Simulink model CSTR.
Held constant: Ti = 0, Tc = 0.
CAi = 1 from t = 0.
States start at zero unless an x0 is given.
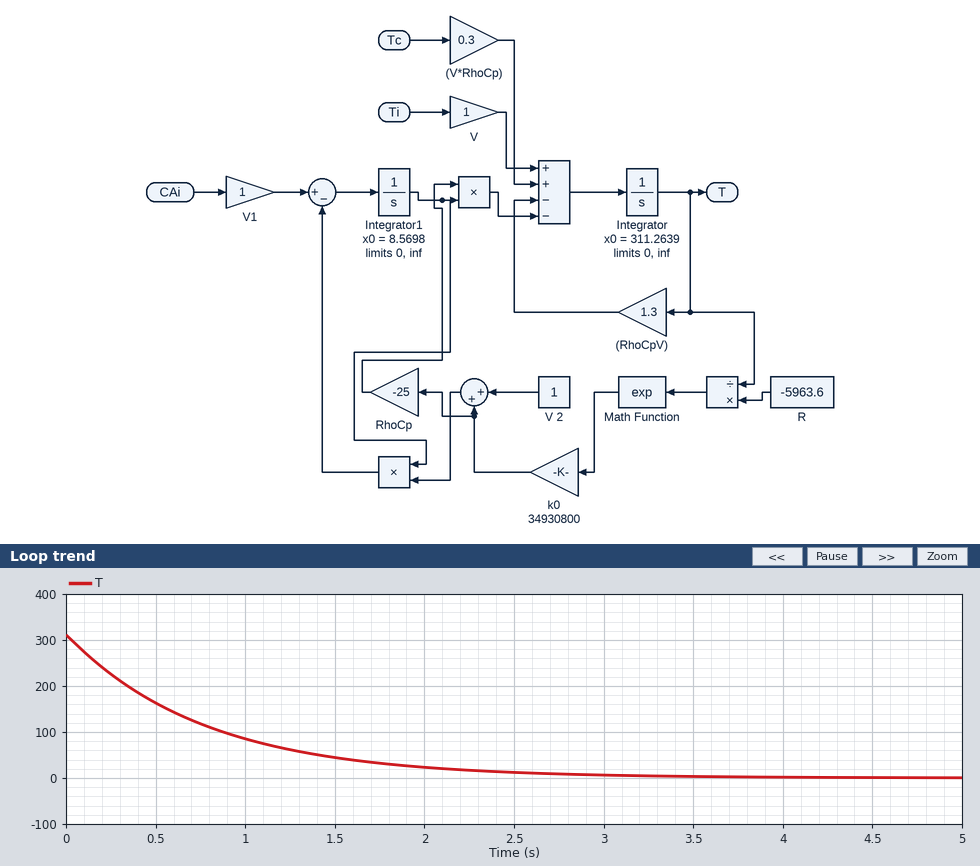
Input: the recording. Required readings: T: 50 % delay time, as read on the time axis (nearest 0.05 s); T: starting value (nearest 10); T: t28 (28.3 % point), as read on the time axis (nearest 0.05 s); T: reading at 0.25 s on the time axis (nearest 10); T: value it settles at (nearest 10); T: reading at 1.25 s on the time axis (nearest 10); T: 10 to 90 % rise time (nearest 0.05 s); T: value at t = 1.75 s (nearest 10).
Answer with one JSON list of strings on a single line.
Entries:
["0.55 s", "310", "0.25 s", "230", "0", "60", "1.70 s", "30"]
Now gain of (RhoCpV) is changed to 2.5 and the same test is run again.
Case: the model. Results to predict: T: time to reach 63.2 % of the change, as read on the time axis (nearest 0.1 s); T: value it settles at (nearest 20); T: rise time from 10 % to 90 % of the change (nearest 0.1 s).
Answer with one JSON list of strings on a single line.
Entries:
["0.4 s", "0", "0.9 s"]
